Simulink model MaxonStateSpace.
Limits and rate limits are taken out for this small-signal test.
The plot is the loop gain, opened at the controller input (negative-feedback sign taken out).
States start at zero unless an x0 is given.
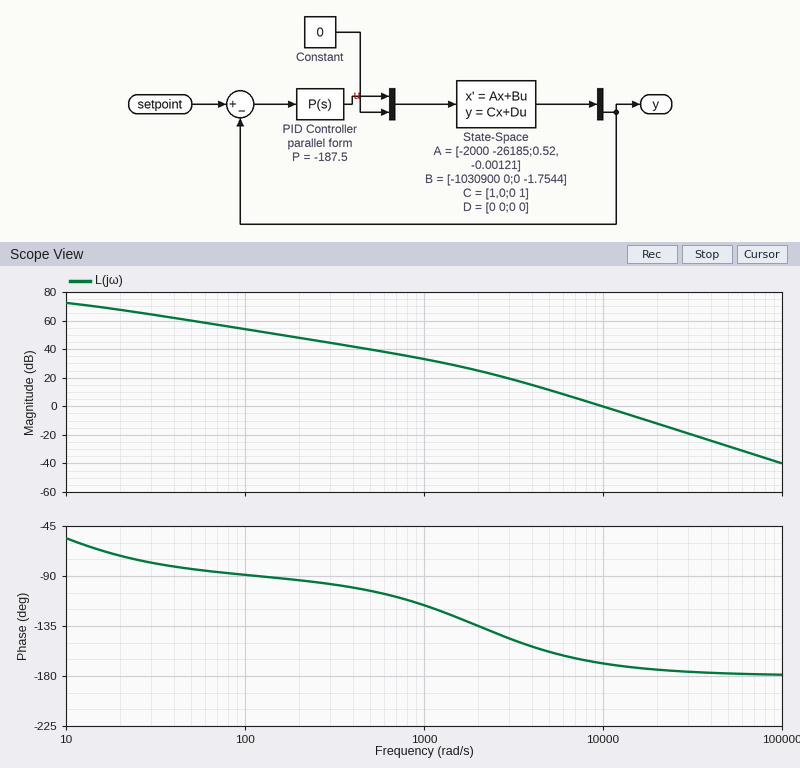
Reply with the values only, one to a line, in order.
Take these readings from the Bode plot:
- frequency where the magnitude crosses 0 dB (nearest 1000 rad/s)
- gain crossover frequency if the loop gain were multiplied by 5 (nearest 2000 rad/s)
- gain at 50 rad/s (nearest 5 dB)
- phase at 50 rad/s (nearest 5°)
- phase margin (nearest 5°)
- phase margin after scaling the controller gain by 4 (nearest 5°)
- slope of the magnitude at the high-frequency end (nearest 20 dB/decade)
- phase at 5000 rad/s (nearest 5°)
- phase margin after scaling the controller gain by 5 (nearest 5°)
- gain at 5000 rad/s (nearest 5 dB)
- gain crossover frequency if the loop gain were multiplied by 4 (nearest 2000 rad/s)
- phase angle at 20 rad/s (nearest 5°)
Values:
10000 rad/s
22000 rad/s
60 dB
-85°
10°
5°
-40 dB/decade
-160°
5°
10 dB
20000 rad/s
-70°
